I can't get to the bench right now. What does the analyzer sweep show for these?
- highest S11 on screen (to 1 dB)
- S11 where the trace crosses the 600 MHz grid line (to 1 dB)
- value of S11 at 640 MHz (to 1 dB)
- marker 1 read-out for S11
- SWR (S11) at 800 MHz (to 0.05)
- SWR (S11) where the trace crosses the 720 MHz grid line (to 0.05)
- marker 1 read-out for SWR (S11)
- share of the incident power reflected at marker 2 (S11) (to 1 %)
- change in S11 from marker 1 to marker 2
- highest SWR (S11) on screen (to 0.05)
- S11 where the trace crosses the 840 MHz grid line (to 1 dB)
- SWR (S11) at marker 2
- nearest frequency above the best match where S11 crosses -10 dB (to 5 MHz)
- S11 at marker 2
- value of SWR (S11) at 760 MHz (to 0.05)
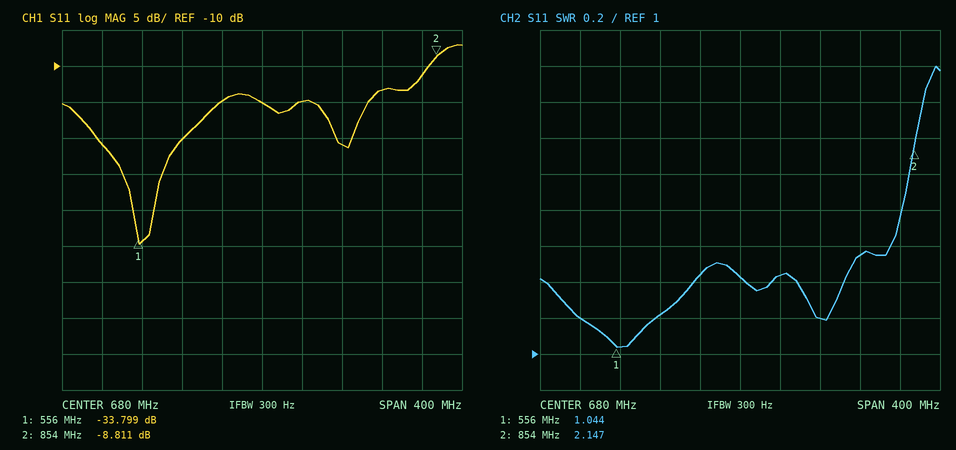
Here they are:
-7 dB
-20 dB
-15 dB
-33.799 dB
1.55
1.45
1.044
13 %
24.988 dB
2.60
-11 dB
2.147
845 MHz
-8.811 dB
1.20
